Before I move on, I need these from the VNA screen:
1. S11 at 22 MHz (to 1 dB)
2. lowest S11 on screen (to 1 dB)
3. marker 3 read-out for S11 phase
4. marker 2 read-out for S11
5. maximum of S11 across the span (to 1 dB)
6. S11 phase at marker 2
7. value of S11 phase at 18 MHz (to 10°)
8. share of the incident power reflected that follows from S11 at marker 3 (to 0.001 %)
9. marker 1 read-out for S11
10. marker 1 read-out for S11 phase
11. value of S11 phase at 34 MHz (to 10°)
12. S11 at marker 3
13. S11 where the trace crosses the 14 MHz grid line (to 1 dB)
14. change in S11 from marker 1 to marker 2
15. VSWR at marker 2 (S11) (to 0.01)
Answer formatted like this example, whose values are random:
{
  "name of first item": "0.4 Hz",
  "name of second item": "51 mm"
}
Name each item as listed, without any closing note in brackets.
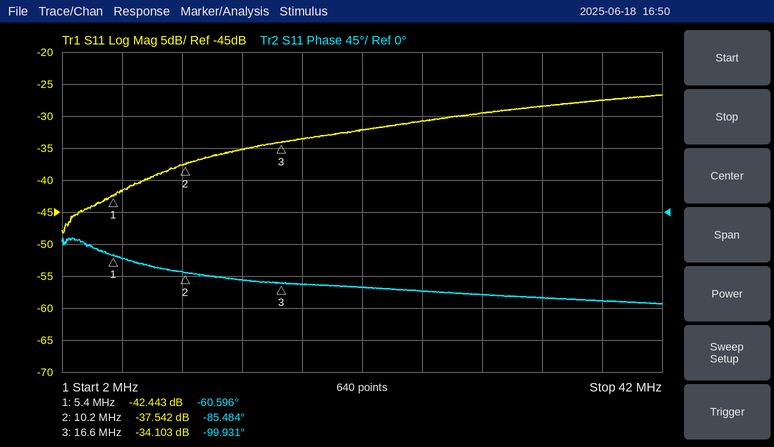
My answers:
{
  "S11 at 22 MHz": "-32 dB",
  "lowest S11 on screen": "-48 dB",
  "marker 3 read-out for S11 phase": "-99.931°",
  "marker 2 read-out for S11": "-37.542 dB",
  "maximum of S11 across the span": "-27 dB",
  "S11 phase at marker 2": "-85.484°",
  "value of S11 phase at 18 MHz": "-100°",
  "share of the incident power reflected that follows from S11 at marker 3": "0.039 %",
  "marker 1 read-out for S11": "-42.443 dB",
  "marker 1 read-out for S11 phase": "-60.596°",
  "value of S11 phase at 34 MHz": "-120°",
  "S11 at marker 3": "-34.103 dB",
  "S11 where the trace crosses the 14 MHz grid line": "-35 dB",
  "change in S11 from marker 1 to marker 2": "4.901 dB",
  "VSWR at marker 2 (S11)": "1.03"
}
